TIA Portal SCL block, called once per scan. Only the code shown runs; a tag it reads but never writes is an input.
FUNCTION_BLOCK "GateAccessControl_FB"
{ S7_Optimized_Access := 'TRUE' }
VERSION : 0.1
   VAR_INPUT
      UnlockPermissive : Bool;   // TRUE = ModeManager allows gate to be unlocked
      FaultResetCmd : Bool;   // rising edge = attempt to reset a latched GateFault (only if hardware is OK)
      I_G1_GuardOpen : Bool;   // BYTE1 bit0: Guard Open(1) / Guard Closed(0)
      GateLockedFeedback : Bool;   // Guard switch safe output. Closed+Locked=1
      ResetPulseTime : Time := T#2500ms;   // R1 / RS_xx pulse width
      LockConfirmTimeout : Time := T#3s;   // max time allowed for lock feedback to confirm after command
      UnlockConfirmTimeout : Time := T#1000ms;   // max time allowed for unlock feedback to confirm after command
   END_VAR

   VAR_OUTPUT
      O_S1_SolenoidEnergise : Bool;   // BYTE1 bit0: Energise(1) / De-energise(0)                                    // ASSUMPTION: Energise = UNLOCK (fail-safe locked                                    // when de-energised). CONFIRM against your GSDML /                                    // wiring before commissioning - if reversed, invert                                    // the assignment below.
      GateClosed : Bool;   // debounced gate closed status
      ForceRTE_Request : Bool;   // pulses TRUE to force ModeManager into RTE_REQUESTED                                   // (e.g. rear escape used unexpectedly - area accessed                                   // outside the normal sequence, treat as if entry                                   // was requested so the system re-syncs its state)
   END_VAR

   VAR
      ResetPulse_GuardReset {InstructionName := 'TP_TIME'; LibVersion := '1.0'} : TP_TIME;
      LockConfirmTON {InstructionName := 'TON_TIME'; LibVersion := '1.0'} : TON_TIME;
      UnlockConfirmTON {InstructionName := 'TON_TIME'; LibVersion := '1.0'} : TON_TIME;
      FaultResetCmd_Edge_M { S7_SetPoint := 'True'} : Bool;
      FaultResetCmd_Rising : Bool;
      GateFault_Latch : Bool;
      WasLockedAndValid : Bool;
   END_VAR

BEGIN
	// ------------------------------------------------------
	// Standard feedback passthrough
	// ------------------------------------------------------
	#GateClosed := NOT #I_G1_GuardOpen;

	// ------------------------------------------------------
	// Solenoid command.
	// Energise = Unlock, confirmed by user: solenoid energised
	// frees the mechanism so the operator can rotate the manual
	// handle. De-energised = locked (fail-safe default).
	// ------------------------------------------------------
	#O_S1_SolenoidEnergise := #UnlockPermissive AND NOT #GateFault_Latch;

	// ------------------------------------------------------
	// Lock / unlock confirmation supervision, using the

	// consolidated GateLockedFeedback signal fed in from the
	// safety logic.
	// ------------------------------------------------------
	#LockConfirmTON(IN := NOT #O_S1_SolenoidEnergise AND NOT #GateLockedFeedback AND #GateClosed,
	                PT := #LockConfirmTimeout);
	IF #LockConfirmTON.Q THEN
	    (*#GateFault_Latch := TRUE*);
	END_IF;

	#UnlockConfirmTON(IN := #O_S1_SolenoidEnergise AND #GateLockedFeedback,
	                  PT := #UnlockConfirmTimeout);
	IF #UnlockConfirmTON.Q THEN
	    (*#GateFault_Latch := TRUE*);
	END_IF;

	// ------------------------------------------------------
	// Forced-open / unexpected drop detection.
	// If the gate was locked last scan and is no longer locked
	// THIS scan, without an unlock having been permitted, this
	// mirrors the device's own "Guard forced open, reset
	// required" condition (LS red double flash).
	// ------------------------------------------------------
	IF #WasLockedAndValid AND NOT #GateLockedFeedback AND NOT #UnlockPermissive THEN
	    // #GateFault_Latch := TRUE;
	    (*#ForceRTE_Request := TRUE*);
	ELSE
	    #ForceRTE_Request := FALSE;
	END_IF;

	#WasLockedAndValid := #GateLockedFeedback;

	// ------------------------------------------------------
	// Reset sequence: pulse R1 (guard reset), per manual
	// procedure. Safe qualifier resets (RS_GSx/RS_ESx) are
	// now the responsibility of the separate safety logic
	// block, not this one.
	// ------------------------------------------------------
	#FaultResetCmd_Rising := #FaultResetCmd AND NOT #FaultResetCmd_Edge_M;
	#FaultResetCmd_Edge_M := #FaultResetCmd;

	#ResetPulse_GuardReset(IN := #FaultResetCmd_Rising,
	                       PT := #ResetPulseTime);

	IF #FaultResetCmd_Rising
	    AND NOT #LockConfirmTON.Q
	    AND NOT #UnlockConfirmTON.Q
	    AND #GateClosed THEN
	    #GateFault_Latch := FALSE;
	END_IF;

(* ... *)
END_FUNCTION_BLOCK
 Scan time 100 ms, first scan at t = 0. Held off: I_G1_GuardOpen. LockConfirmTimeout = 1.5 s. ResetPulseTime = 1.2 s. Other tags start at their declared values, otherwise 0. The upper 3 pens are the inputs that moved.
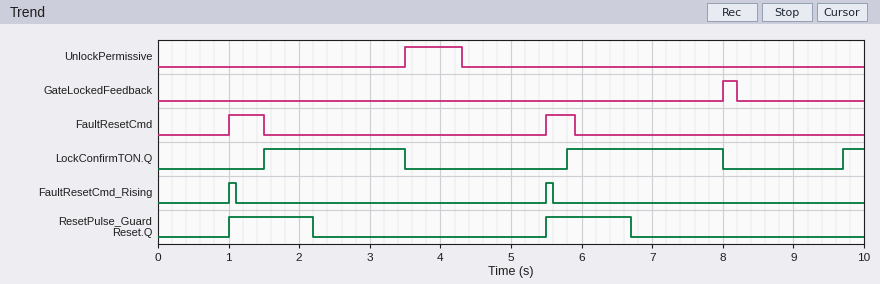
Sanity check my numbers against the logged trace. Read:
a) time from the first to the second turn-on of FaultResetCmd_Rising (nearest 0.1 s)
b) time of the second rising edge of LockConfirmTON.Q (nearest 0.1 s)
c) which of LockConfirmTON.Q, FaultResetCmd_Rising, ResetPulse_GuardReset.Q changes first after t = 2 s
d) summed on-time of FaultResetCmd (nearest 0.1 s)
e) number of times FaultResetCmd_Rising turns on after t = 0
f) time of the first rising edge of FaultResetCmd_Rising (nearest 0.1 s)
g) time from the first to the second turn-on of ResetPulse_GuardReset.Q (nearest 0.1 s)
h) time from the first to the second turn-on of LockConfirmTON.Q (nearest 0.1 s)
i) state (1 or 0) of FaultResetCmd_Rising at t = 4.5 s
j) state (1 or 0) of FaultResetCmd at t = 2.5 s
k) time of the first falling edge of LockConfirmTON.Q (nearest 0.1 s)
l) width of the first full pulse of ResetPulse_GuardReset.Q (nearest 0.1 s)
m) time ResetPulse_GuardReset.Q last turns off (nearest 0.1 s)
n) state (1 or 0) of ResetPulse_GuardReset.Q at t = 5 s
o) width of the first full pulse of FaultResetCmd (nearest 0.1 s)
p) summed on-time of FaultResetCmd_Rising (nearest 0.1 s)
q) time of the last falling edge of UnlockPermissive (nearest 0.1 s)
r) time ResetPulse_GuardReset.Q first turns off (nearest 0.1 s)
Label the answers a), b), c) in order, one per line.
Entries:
a) 4.5 s
b) 5.8 s
c) ResetPulse_GuardReset.Q
d) 0.9 s
e) 2
f) 1.0 s
g) 4.5 s
h) 4.3 s
i) 0
j) 0
k) 3.5 s
l) 1.2 s
m) 6.7 s
n) 0
o) 0.5 s
p) 0.2 s
q) 4.3 s
r) 2.2 s
